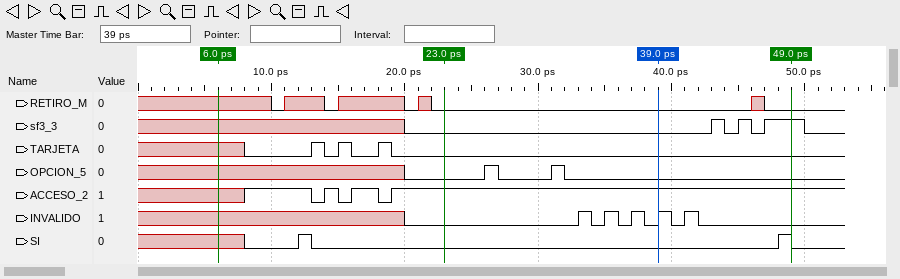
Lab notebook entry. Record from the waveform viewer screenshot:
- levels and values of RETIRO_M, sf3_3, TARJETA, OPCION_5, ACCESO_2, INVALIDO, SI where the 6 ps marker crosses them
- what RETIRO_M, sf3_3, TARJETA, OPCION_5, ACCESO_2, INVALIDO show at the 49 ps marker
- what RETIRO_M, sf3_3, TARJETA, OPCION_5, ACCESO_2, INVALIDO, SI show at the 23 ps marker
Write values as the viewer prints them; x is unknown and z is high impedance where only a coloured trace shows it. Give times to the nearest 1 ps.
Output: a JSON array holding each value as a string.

["RETIRO_M=x, sf3_3=x, TARJETA=x, OPCION_5=x, ACCESO_2=x, INVALIDO=x, SI=x", "RETIRO_M=0, sf3_3=1, TARJETA=0, OPCION_5=0, ACCESO_2=1, INVALIDO=0", "RETIRO_M=0, sf3_3=0, TARJETA=0, OPCION_5=0, ACCESO_2=1, INVALIDO=0, SI=0"]
